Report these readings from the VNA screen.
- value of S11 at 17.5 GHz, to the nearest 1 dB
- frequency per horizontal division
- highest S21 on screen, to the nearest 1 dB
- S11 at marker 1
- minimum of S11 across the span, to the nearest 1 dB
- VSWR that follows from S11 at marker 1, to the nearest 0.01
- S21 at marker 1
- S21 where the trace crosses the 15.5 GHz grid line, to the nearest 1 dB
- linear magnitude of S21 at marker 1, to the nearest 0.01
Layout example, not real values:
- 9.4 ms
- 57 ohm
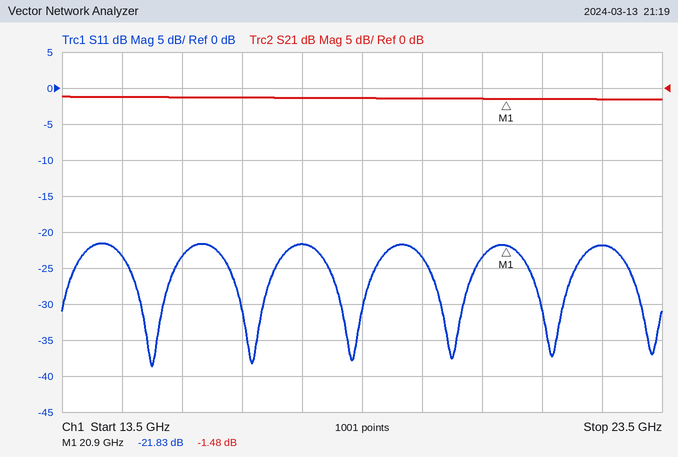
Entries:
- -22 dB
- 1 GHz
- -1 dB
- -21.83 dB
- -39 dB
- 1.18
- -1.48 dB
- -1 dB
- 0.84
